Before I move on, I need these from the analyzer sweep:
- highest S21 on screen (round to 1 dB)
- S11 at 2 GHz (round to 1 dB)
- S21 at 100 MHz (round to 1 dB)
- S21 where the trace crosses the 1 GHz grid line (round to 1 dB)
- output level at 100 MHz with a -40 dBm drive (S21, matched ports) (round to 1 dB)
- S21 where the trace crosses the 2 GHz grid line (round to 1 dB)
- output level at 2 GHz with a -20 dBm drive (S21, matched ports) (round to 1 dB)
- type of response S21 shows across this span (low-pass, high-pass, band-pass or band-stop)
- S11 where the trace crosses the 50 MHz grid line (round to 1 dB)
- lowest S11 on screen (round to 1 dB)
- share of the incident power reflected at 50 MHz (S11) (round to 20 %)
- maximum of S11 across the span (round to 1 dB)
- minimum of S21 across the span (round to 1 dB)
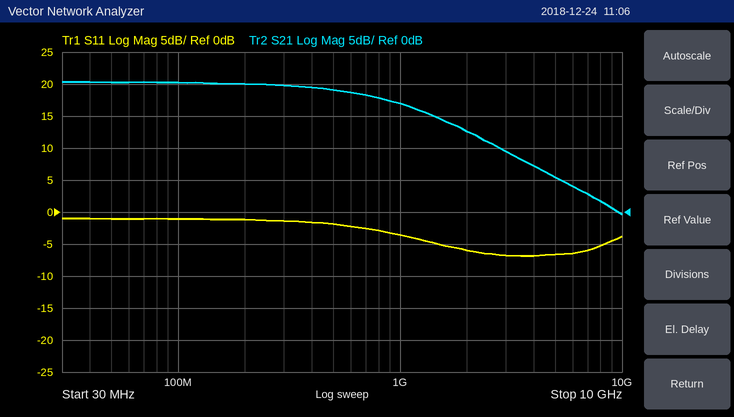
20 dB
-6 dB
20 dB
17 dB
-20 dBm
13 dB
-7 dBm
low-pass
-1 dB
-7 dB
80 %
-1 dB
0 dB
